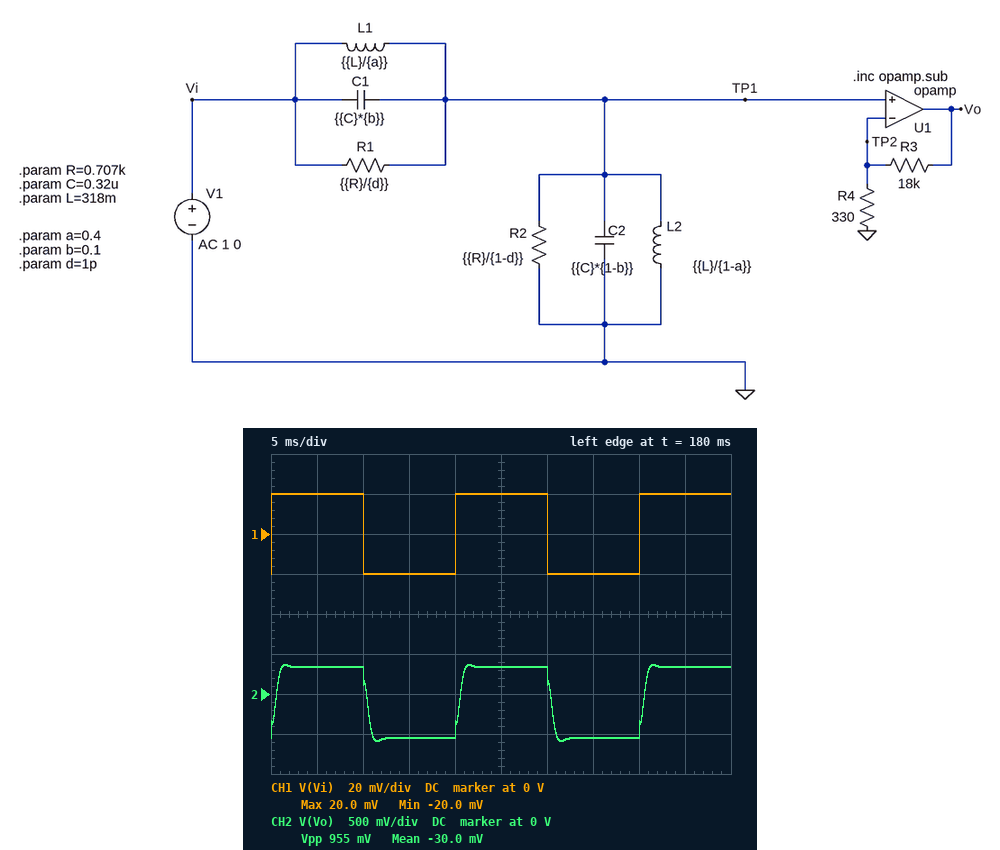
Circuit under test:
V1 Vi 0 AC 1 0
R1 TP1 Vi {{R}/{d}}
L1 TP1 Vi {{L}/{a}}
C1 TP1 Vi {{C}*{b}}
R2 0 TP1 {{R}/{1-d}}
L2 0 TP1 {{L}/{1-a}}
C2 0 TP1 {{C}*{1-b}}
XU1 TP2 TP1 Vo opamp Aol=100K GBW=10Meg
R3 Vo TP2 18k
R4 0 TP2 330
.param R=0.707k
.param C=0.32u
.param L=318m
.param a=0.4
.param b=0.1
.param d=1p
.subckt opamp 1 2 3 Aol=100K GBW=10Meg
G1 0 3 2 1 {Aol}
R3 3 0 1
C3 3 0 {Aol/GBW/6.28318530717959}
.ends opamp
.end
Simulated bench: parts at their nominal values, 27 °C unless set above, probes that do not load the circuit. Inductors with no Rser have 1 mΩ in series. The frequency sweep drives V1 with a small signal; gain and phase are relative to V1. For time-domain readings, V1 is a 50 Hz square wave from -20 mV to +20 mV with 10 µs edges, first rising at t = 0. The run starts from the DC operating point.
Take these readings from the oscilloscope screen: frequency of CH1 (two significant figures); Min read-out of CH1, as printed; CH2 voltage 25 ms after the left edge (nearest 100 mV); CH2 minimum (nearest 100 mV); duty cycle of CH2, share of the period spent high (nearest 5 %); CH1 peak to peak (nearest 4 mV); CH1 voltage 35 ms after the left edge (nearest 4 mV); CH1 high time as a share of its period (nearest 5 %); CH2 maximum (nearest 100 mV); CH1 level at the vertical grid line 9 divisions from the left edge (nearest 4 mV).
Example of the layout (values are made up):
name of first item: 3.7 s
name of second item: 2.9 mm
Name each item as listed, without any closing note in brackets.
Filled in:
frequency of CH1: 50 Hz
Min read-out of CH1, as printed: -20.0 mV
CH2 voltage 25 ms after the left edge: 300 mV
CH2 minimum: -600 mV
duty cycle of CH2, share of the period spent high: 50 %
CH1 peak to peak: 40 mV
CH1 voltage 35 ms after the left edge: -20 mV
CH1 high time as a share of its period: 50 %
CH2 maximum: 400 mV
CH1 level at the vertical grid line 9 divisions from the left edge: 20 mV
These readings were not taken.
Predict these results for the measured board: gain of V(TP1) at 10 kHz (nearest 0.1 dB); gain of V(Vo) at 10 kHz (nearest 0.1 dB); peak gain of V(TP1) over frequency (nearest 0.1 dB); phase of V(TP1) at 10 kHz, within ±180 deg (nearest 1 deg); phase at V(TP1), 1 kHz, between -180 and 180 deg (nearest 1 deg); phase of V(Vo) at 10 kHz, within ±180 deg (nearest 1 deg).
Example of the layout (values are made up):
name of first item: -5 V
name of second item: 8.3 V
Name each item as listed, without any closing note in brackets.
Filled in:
gain of V(TP1) at 10 kHz: -20.1 dB
gain of V(Vo) at 10 kHz: 14.8 dB
peak gain of V(TP1) over frequency: -8.0 dB
phase of V(TP1) at 10 kHz, within ±180 deg: 4 deg
phase at V(TP1), 1 kHz, between -180 and 180 deg: 43 deg
phase of V(Vo) at 10 kHz, within ±180 deg: 1 deg
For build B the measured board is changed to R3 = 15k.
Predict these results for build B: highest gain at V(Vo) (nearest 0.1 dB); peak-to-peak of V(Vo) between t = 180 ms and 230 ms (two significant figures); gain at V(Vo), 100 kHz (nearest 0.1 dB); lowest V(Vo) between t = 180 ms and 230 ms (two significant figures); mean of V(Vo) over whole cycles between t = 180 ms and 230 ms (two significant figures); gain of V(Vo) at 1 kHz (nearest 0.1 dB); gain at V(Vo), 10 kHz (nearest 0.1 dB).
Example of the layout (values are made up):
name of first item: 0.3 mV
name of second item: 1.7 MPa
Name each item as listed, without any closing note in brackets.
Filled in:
highest gain at V(Vo): 25.4 dB
peak-to-peak of V(Vo) between t = 180 ms and 230 ms: 800 mV
gain at V(Vo), 100 kHz: 12.5 dB
lowest V(Vo) between t = 180 ms and 230 ms: -490 mV
mean of V(Vo) over whole cycles between t = 180 ms and 230 ms: -93 mV
gain of V(Vo) at 1 kHz: -34.2 dB
gain at V(Vo), 10 kHz: 13.2 dB
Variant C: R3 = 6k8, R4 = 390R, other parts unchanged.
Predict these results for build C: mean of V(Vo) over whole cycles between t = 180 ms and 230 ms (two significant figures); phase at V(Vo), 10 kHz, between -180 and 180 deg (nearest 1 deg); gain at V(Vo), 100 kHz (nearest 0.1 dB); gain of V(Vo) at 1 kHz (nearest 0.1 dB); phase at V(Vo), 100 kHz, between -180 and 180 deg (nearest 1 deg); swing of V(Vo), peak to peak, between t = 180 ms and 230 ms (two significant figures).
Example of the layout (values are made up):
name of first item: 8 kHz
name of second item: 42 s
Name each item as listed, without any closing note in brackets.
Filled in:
mean of V(Vo) over whole cycles between t = 180 ms and 230 ms: -37 mV
phase at V(Vo), 10 kHz, between -180 and 180 deg: 3 deg
gain at V(Vo), 100 kHz: 5.2 dB
gain of V(Vo) at 1 kHz: -42.2 dB
phase at V(Vo), 100 kHz, between -180 and 180 deg: -10 deg
swing of V(Vo), peak to peak, between t = 180 ms and 230 ms: 320 mV
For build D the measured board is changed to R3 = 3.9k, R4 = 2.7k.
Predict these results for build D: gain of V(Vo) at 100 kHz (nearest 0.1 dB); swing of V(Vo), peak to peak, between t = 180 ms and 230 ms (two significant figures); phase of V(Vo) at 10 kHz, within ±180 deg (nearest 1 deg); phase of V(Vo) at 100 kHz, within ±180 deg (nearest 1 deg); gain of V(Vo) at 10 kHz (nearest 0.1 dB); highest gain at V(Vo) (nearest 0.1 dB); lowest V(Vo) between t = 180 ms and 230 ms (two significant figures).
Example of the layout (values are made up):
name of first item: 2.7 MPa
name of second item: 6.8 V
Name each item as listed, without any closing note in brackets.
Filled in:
gain of V(Vo) at 100 kHz: -12.2 dB
swing of V(Vo), peak to peak, between t = 180 ms and 230 ms: 42 mV
phase of V(Vo) at 10 kHz, within ±180 deg: 4 deg
phase of V(Vo) at 100 kHz, within ±180 deg: -1 deg
gain of V(Vo) at 10 kHz: -12.3 dB
highest gain at V(Vo): -0.2 dB
lowest V(Vo) between t = 180 ms and 230 ms: -26 mV
